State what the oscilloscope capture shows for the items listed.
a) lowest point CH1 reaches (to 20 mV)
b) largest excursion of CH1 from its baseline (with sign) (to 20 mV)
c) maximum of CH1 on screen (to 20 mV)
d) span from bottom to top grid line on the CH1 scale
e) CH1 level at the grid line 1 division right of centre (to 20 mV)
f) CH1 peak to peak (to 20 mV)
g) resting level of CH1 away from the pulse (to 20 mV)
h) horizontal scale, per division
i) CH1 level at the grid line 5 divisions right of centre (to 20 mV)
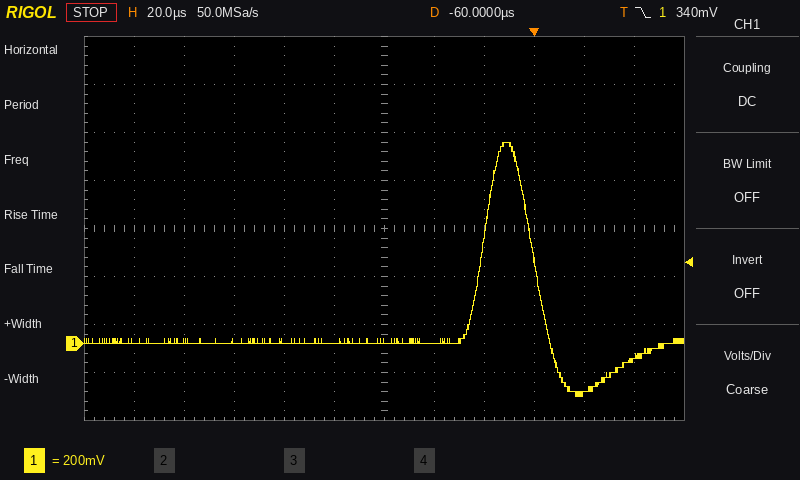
-220 mV
+840 mV
840 mV
1.6 V
0 mV
1.06 V
0 mV
20 µs
-60 mV
